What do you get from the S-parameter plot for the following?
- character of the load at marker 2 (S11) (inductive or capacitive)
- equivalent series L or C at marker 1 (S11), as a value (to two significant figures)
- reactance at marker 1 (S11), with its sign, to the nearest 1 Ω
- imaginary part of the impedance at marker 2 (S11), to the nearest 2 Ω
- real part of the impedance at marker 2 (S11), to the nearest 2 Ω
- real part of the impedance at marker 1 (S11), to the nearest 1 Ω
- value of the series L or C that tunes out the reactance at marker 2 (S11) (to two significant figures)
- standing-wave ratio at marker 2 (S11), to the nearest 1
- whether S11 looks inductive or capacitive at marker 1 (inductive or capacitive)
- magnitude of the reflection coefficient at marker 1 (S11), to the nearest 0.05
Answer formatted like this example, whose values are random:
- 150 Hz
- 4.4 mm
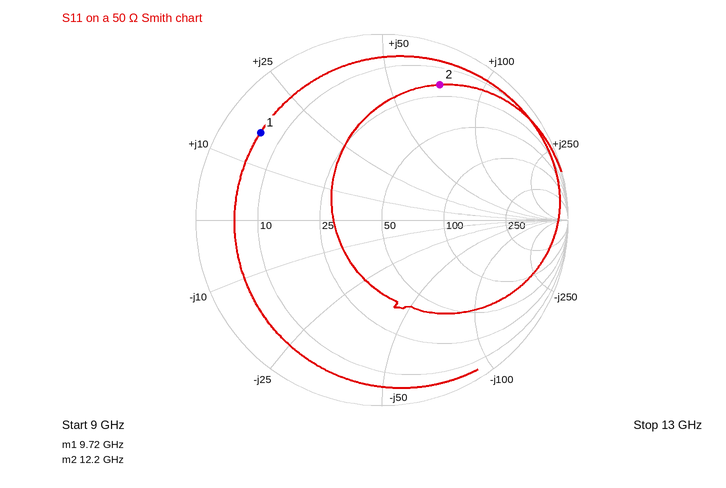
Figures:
- inductive
- 260 pH
- +16 Ω
- +72 Ω
- 18 Ω
- 6 Ω
- 180 fF
- 9
- inductive
- 0.80
